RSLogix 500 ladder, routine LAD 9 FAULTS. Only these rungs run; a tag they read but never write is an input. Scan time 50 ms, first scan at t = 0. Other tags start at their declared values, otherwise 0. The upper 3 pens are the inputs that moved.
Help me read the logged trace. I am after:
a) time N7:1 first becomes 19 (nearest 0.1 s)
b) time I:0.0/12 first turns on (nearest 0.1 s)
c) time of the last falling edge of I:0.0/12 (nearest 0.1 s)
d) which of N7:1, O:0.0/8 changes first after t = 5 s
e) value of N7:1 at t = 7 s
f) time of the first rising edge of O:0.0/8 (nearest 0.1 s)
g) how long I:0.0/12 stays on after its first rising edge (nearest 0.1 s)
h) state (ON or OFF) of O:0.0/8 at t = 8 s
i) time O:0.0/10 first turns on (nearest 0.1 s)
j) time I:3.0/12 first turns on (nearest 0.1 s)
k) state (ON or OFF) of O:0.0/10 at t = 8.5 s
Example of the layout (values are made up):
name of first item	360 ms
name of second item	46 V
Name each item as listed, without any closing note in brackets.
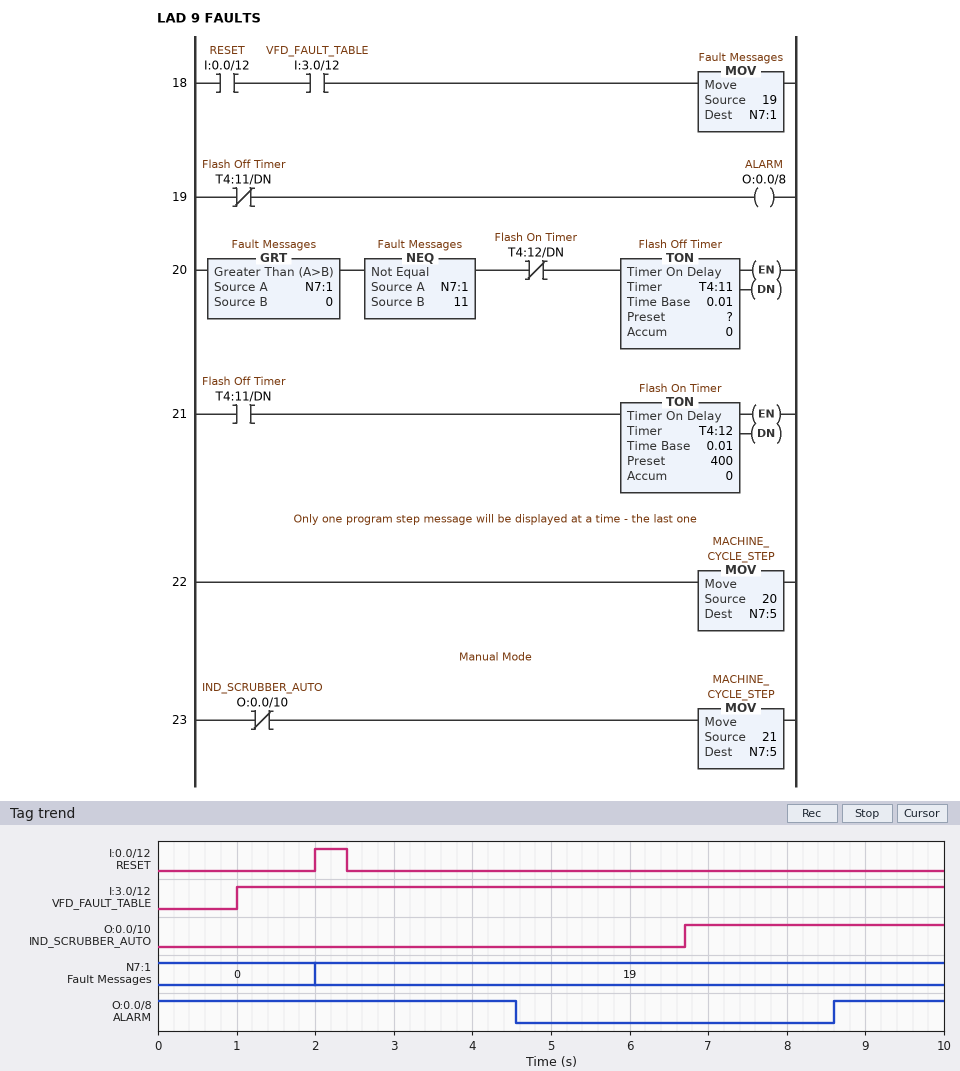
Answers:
time N7:1 first becomes 19	2.0 s
time I:0.0/12 first turns on	2.0 s
time of the last falling edge of I:0.0/12	2.4 s
which of N7:1, O:0.0/8 changes first after t = 5 s	O:0.0/8
value of N7:1 at t = 7 s	19
time of the first rising edge of O:0.0/8	8.6 s
how long I:0.0/12 stays on after its first rising edge	0.4 s
state (ON or OFF) of O:0.0/8 at t = 8 s	OFF
time O:0.0/10 first turns on	6.7 s
time I:3.0/12 first turns on	1.0 s
state (ON or OFF) of O:0.0/10 at t = 8.5 s	ON
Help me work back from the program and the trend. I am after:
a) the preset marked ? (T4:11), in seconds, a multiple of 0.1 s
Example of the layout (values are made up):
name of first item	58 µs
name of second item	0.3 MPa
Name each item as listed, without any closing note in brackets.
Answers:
the preset marked ? (T4:11), in seconds, a multiple of 0.1 s	2.5 s
